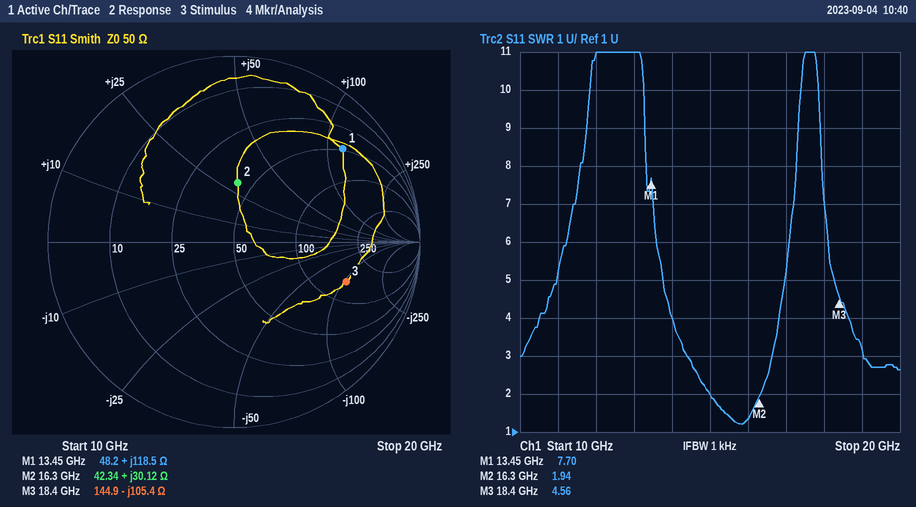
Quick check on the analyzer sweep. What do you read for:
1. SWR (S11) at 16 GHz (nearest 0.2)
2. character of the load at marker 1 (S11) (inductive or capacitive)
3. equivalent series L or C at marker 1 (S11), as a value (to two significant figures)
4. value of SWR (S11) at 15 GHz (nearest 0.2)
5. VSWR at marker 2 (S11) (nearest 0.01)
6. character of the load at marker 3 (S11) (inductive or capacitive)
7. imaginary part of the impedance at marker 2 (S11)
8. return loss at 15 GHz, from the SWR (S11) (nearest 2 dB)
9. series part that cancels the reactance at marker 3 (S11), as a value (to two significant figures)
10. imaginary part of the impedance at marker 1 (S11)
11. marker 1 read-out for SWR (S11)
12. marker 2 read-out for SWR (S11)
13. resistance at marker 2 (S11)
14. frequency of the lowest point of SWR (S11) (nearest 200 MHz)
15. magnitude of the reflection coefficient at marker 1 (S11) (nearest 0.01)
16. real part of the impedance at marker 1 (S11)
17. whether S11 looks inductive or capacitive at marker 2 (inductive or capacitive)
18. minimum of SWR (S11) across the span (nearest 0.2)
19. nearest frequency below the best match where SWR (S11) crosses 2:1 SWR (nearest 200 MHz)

1.4
inductive
1.4 nH
2.0
1.94
capacitive
+30.12 Ω
10 dB
910 pH
+118.5 Ω
7.70
1.94
42.34 Ω
15.8 GHz
0.77
48.2 Ω
inductive
1.2
15.0 GHz
